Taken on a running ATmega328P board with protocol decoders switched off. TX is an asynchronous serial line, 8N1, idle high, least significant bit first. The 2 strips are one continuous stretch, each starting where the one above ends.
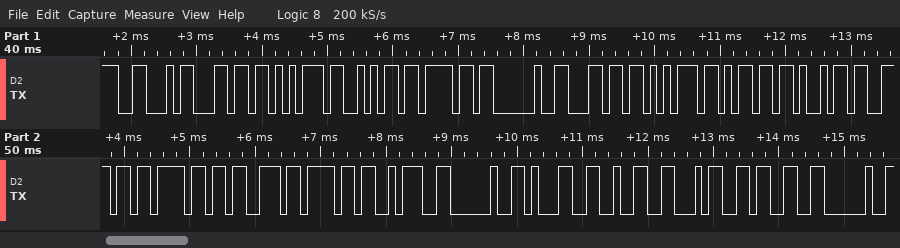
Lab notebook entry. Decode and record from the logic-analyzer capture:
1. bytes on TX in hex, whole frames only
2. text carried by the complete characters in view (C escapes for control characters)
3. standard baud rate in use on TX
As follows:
46 6C 75 6A 6F 20 6C 75 6D 69 6E 6F 73 6F 3A 20 31 32 34 33 20
"Flujo luminoso: 1243 "
9600 baud
